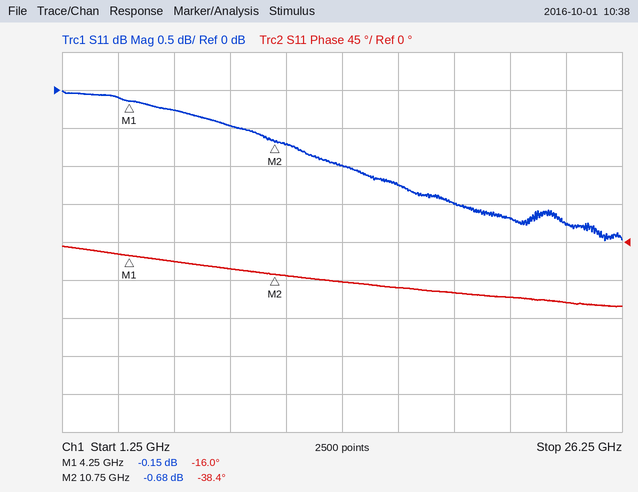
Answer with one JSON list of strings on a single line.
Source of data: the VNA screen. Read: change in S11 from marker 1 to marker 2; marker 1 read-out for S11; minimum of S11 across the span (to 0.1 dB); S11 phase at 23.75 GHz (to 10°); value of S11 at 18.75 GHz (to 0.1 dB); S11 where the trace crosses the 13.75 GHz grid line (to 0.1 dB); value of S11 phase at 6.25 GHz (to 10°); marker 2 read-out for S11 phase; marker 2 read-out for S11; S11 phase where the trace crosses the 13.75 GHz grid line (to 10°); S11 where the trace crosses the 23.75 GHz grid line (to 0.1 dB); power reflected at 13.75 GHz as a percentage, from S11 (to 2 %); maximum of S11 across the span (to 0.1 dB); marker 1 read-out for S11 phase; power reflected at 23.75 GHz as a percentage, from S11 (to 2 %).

["-0.53 dB", "-0.15 dB", "-2.0 dB", "-70°", "-1.5 dB", "-1.0 dB", "-20°", "-38.4°", "-0.68 dB", "-50°", "-1.8 dB", "80 %", "0.0 dB", "-16.0°", "66 %"]
